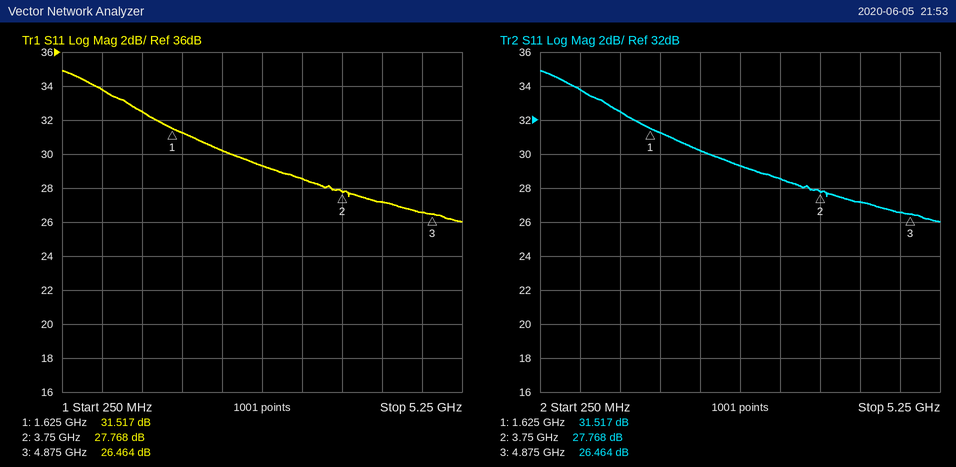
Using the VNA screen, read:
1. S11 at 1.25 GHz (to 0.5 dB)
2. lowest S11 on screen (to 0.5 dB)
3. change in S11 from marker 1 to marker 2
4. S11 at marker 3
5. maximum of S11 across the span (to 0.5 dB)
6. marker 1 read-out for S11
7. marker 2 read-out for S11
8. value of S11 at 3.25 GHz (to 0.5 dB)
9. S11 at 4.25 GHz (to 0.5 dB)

32.5 dB
26.0 dB
-3.749 dB
26.464 dB
35.0 dB
31.517 dB
27.768 dB
28.5 dB
27.0 dB
